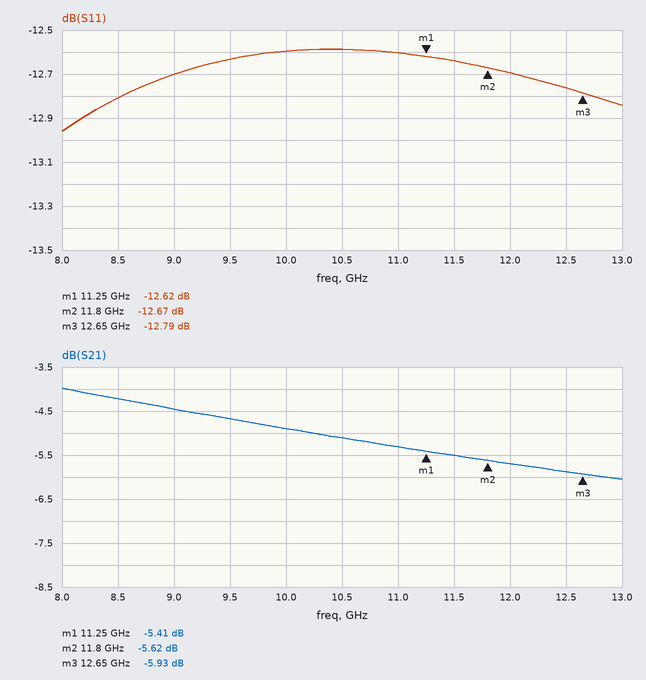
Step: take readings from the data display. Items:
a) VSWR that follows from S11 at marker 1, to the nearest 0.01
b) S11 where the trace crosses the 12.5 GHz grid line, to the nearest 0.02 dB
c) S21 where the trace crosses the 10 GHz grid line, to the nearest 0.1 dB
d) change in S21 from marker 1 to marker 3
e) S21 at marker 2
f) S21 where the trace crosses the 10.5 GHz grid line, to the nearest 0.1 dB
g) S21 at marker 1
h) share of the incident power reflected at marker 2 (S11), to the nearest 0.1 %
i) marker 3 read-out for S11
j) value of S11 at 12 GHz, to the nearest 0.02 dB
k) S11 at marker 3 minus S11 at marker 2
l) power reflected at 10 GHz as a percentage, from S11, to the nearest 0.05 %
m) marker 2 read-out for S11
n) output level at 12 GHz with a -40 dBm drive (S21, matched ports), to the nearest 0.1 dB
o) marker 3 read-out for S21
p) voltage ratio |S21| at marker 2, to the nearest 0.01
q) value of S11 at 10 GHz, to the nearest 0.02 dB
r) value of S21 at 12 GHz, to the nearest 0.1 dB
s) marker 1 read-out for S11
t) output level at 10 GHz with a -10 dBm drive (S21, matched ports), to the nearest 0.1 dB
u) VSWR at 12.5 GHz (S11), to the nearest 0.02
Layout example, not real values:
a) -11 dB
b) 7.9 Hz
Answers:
a) 1.61
b) -12.76 dB
c) -4.9 dB
d) -0.52 dB
e) -5.62 dB
f) -5.1 dB
g) -5.41 dB
h) 5.4 %
i) -12.79 dB
j) -12.70 dB
k) -0.12 dB
l) 5.50 %
m) -12.67 dB
n) -45.7 dBm
o) -5.93 dB
p) 0.52
q) -12.60 dB
r) -5.7 dB
s) -12.62 dB
t) -14.9 dBm
u) 1.60
